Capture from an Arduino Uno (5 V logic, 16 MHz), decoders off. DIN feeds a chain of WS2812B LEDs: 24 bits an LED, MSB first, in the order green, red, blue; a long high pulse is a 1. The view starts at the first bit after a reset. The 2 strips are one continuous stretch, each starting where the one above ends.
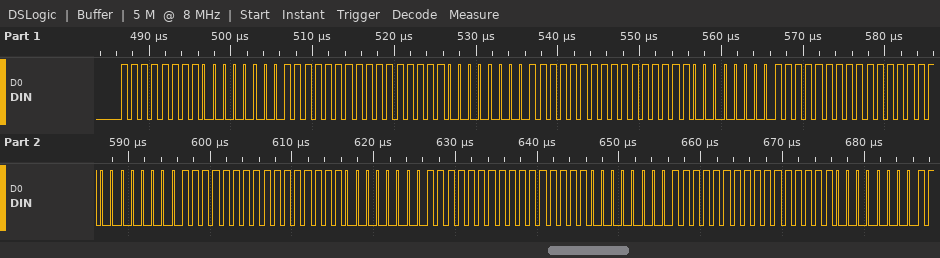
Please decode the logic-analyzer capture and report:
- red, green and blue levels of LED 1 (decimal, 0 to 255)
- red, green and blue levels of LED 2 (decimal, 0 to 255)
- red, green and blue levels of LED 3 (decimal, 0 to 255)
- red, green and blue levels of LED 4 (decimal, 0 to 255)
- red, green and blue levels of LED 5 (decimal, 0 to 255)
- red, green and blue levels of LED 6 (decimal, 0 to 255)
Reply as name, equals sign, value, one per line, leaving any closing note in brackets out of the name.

red, green and blue levels of LED 1 = 0, 255, 255
red, green and blue levels of LED 2 = 0, 255, 255
red, green and blue levels of LED 3 = 0, 255, 255
red, green and blue levels of LED 4 = 0, 255, 255
red, green and blue levels of LED 5 = 0, 255, 255
red, green and blue levels of LED 6 = 0, 255, 255
